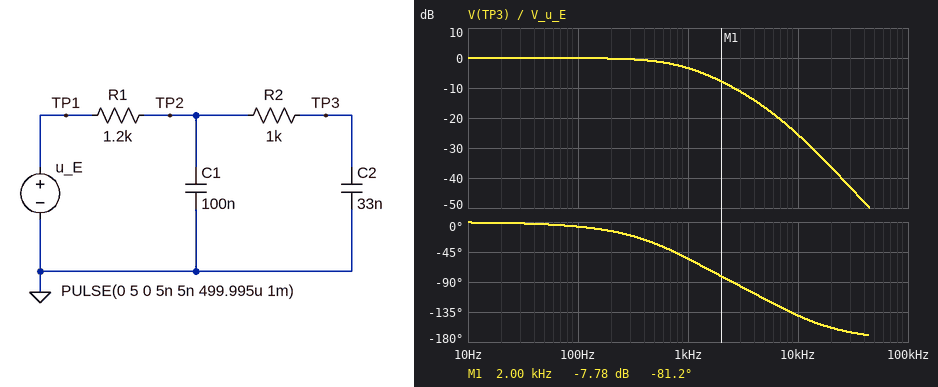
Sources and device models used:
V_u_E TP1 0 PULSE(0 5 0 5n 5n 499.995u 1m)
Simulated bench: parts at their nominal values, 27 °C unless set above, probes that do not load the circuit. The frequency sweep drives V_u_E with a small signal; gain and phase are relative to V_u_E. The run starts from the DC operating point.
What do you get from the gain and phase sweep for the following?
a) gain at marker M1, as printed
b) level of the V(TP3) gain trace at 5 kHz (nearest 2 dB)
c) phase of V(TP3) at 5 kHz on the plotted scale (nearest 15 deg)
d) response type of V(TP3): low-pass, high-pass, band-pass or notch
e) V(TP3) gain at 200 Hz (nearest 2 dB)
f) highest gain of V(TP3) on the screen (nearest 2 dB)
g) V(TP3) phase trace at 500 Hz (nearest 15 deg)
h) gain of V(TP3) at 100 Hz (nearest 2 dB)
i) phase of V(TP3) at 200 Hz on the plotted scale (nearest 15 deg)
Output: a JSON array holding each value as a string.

["-7.78 dB", "-16 dB", "-120 deg", "low-pass", "0 dB", "0 dB", "-30 deg", "0 dB", "-15 deg"]
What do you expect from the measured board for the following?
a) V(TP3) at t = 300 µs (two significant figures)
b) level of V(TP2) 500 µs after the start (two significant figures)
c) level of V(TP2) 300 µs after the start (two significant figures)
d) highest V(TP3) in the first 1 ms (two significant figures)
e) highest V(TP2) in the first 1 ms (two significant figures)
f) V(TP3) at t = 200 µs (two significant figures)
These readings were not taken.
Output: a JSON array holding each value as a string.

["4.0 V", "4.8 V", "4.2 V", "4.7 V", "4.8 V", "3.2 V"]
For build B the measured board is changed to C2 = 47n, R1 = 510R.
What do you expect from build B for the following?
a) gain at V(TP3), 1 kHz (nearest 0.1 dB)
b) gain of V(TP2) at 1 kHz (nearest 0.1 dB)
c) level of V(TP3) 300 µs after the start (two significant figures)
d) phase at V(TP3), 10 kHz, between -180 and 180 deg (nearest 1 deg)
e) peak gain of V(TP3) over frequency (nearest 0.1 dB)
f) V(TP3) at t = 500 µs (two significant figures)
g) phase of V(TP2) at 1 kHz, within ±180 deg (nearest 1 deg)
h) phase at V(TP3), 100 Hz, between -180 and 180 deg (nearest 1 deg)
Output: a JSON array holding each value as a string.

["-1.5 dB", "-1.1 dB", "4.7 V", "-138 deg", "0 dB", "5.0 V", "-24 deg", "-4 deg"]
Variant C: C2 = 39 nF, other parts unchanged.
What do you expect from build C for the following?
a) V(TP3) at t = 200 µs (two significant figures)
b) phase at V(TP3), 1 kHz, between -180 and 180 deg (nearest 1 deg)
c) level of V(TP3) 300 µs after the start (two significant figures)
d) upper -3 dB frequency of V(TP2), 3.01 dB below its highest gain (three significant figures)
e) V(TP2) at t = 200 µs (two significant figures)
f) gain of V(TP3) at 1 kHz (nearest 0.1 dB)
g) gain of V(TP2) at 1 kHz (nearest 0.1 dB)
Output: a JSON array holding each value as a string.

["3.1 V", "-58 deg", "3.9 V", "909 Hz", "3.5 V", "-3.7 dB", "-3.4 dB"]
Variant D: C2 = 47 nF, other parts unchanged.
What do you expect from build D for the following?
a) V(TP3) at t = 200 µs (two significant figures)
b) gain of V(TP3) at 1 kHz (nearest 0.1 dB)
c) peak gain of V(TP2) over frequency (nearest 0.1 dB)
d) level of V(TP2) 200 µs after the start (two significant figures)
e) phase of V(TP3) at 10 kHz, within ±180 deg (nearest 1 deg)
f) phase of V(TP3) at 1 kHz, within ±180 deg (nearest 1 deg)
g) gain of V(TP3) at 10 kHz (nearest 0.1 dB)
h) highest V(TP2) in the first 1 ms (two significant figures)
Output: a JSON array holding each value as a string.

["2.9 V", "-4.1 dB", "0 dB", "3.4 V", "-147 deg", "-61 deg", "-28.1 dB", "4.7 V"]
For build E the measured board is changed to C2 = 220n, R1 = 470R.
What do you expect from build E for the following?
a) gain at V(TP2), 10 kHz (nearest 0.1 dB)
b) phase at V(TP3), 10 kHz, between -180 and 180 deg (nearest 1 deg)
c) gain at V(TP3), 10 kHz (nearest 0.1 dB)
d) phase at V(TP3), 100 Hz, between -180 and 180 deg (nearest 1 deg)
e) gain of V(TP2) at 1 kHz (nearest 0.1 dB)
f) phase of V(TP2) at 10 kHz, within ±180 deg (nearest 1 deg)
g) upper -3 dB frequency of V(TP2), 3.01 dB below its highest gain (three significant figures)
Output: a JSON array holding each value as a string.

["-10.4 dB", "-150 deg", "-33.3 dB", "-13 deg", "-3.0 dB", "-64 deg", "1.02 kHz"]
